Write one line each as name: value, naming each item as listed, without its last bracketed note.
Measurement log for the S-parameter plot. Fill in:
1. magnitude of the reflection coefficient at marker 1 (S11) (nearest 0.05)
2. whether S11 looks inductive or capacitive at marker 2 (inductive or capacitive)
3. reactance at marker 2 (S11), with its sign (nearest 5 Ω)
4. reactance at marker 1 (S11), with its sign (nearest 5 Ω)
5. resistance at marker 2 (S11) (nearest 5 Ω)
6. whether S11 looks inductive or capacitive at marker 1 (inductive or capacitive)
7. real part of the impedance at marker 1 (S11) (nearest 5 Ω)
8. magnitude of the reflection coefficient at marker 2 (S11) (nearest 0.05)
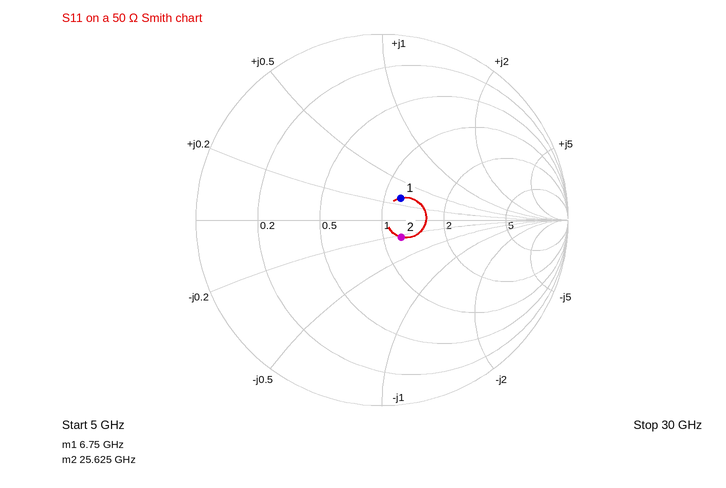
magnitude of the reflection coefficient at marker 1 (S11): 0.15
whether S11 looks inductive or capacitive at marker 2: capacitive
reactance at marker 2 (S11), with its sign: -10 Ω
reactance at marker 1 (S11), with its sign: +15 Ω
resistance at marker 2 (S11): 60 Ω
whether S11 looks inductive or capacitive at marker 1: inductive
real part of the impedance at marker 1 (S11): 60 Ω
magnitude of the reflection coefficient at marker 2 (S11): 0.15
